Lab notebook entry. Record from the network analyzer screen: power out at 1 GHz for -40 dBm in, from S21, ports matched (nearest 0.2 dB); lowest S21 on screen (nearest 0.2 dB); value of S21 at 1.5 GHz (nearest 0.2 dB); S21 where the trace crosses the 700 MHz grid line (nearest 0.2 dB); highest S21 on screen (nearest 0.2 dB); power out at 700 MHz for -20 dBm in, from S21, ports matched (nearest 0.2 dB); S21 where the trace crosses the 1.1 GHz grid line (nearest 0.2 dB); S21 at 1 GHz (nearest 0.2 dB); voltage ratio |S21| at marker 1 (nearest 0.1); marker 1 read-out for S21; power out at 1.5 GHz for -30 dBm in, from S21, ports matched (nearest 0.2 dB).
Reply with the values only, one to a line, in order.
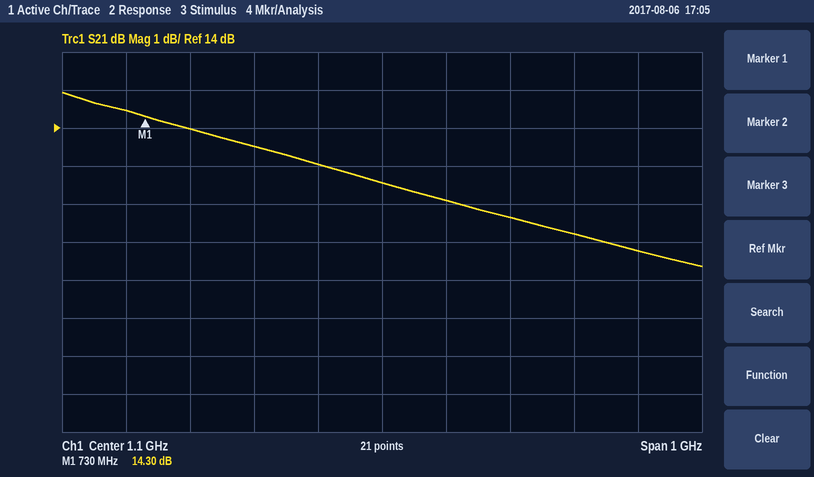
-27.0 dBm
10.4 dB
10.8 dB
14.4 dB
15.0 dB
-5.6 dBm
12.6 dB
13.0 dB
5.2
14.30 dB
-19.2 dBm
